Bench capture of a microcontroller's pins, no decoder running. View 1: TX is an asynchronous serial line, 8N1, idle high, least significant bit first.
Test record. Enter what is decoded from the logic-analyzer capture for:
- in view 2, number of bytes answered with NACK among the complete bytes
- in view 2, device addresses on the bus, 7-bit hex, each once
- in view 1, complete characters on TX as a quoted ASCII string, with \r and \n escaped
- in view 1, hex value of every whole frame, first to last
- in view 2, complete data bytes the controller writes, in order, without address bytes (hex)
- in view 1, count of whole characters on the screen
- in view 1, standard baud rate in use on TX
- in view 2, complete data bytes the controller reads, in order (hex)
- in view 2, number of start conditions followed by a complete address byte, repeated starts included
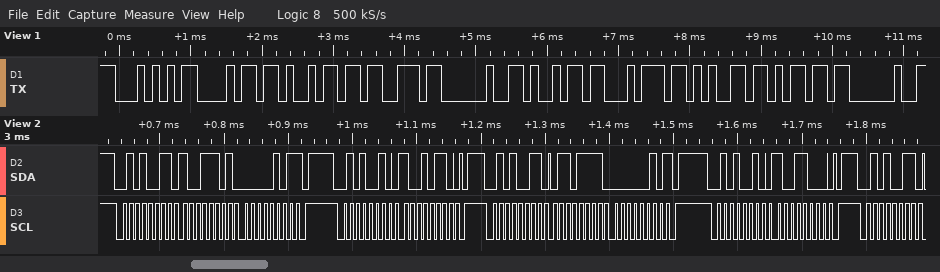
2
0x29
"This item "
0x54 0x68 0x69 0x73 0x20 0x69 0x74 0x65 0x6D 0x20
96 98
10
9600 baud
9D 05 6F 02
5
